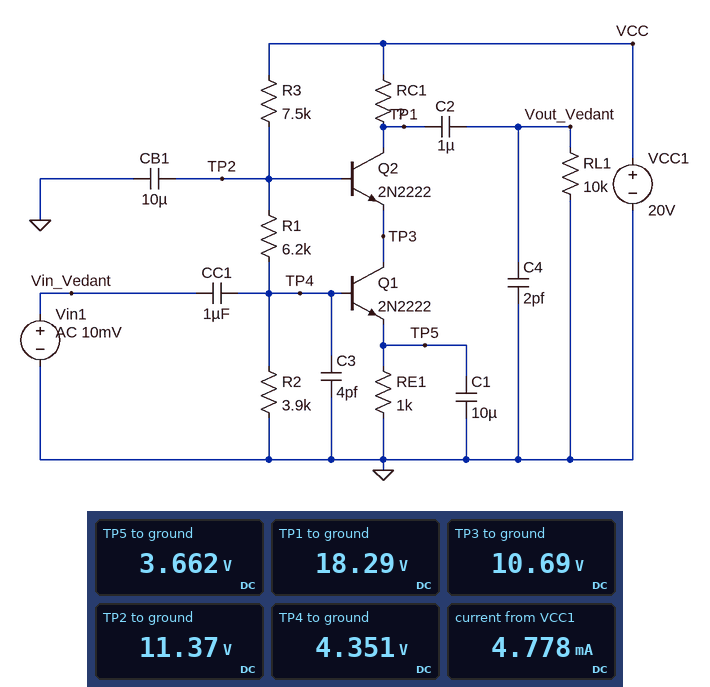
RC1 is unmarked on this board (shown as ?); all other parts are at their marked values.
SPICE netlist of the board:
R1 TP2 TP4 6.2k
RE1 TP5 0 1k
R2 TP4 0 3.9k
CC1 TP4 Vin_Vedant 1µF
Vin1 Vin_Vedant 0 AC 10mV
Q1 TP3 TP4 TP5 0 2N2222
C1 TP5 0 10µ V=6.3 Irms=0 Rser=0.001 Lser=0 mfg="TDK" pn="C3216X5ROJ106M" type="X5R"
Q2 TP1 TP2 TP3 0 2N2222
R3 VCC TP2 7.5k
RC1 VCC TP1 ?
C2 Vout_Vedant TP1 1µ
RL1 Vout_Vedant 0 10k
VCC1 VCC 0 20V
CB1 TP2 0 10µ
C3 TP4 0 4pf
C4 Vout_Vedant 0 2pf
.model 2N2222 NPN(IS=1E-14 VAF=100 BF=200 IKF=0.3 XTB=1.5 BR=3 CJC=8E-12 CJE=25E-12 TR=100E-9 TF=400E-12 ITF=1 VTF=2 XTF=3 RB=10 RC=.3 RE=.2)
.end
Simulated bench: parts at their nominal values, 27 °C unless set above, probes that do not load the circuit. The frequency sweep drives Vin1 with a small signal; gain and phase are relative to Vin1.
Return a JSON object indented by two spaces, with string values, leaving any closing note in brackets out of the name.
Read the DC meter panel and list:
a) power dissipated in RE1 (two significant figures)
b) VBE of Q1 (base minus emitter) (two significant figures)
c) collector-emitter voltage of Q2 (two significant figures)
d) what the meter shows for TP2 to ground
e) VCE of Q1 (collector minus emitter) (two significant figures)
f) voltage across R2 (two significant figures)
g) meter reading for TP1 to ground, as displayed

{
  "power dissipated in RE1": "13 mW",
  "VBE of Q1 (base minus emitter)": "690 mV",
  "collector-emitter voltage of Q2": "7.6 V",
  "what the meter shows for TP2 to ground": "11.37 V",
  "VCE of Q1 (collector minus emitter)": "7.0 V",
  "voltage across R2": "4.4 V",
  "meter reading for TP1 to ground, as displayed": "18.29 V"
}
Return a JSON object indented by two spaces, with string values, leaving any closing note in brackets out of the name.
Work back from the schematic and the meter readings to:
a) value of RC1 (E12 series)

{
  "value of RC1": "470 Ω"
}
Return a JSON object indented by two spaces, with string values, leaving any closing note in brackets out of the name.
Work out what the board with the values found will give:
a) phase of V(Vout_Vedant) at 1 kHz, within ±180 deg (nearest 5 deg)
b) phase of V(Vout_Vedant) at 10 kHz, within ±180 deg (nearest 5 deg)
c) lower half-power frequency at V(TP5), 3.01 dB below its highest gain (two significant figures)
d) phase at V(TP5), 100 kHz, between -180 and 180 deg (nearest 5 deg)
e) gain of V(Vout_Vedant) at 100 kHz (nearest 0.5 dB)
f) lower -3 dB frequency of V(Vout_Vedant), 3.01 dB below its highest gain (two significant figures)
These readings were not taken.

{
  "phase of V(Vout_Vedant) at 1 kHz, within ±180 deg": "-110 deg",
  "phase of V(Vout_Vedant) at 10 kHz, within ±180 deg": "-165 deg",
  "lower half-power frequency at V(TP5), 3.01 dB below its highest gain": "62 Hz",
  "phase at V(TP5), 100 kHz, between -180 and 180 deg": "-90 deg",
  "gain of V(Vout_Vedant) at 100 kHz": "35.5 dB",
  "lower -3 dB frequency of V(Vout_Vedant), 3.01 dB below its highest gain": "2.3 kHz"
}
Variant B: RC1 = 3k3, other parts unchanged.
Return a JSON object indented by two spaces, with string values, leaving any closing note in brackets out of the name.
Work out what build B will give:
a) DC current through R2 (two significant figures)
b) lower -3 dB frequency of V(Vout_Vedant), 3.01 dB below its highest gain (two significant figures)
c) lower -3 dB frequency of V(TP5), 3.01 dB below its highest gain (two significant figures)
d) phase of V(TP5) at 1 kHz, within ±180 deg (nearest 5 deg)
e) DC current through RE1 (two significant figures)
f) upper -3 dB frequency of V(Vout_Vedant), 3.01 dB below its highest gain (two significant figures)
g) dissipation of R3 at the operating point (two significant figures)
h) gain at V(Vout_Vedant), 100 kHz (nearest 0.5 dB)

{
  "DC current through R2": "1.0 mA",
  "lower -3 dB frequency of V(Vout_Vedant), 3.01 dB below its highest gain": "2.0 kHz",
  "lower -3 dB frequency of V(TP5), 3.01 dB below its highest gain": "81 Hz",
  "phase of V(TP5) at 1 kHz, within ±180 deg": "-20 deg",
  "DC current through RE1": "3.3 mA",
  "upper -3 dB frequency of V(Vout_Vedant), 3.01 dB below its highest gain": "570 kHz",
  "dissipation of R3 at the operating point": "12 mW",
  "gain at V(Vout_Vedant), 100 kHz": "23.5 dB"
}
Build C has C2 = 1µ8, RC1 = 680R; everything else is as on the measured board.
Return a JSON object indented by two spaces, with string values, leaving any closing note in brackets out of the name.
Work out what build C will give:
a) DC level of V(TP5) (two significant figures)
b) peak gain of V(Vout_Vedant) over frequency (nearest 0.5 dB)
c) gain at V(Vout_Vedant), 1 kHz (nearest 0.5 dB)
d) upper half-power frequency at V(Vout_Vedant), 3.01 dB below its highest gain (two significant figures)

{
  "DC level of V(TP5)": "3.7 V",
  "peak gain of V(Vout_Vedant) over frequency": "38.5 dB",
  "gain at V(Vout_Vedant), 1 kHz": "30.5 dB",
  "upper half-power frequency at V(Vout_Vedant), 3.01 dB below its highest gain": "39 MHz"
}
